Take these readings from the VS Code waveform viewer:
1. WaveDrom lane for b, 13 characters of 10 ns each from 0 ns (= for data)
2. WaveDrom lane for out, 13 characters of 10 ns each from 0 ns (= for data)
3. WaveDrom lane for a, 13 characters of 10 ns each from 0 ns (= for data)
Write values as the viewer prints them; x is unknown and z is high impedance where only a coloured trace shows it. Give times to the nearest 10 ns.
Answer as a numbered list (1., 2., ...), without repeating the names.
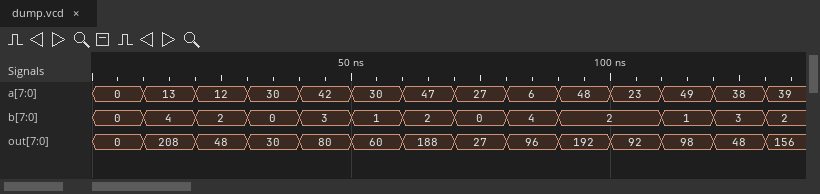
1. {name: 'b', wave: '==========.==', data: '0 4 2 0 3 1 2 0 4 2 1 3'}
2. {name: 'out', wave: '=============', data: '0 208 48 30 80 60 188 27 96 192 92 98 48'}
3. {name: 'a', wave: '=============', data: '0 13 12 30 42 30 47 27 6 48 23 49 38'}
